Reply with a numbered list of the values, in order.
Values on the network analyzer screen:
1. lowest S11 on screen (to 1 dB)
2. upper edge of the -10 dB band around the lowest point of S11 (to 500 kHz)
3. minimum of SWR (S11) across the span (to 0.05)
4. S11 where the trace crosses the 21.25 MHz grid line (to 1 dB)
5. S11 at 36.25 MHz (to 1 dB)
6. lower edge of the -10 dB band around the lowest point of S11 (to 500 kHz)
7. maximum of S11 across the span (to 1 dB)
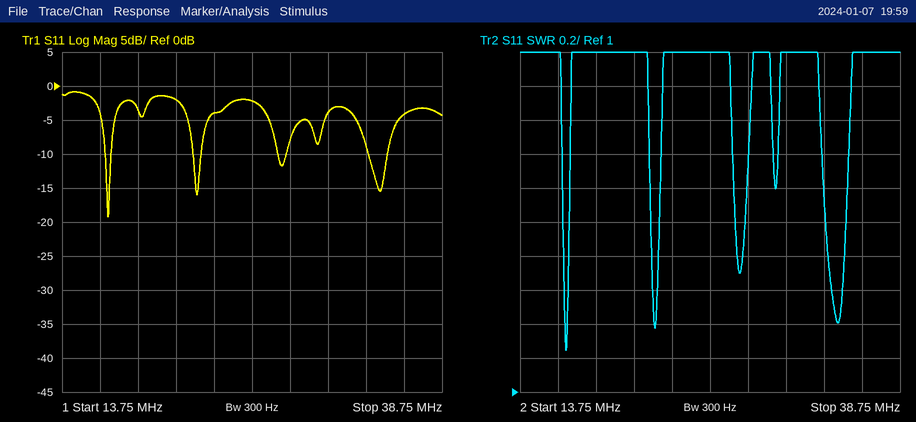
1. -19 dB
2. 17.0 MHz
3. 1.25
4. -2 dB
5. -4 dB
6. 16.5 MHz
7. -1 dB
